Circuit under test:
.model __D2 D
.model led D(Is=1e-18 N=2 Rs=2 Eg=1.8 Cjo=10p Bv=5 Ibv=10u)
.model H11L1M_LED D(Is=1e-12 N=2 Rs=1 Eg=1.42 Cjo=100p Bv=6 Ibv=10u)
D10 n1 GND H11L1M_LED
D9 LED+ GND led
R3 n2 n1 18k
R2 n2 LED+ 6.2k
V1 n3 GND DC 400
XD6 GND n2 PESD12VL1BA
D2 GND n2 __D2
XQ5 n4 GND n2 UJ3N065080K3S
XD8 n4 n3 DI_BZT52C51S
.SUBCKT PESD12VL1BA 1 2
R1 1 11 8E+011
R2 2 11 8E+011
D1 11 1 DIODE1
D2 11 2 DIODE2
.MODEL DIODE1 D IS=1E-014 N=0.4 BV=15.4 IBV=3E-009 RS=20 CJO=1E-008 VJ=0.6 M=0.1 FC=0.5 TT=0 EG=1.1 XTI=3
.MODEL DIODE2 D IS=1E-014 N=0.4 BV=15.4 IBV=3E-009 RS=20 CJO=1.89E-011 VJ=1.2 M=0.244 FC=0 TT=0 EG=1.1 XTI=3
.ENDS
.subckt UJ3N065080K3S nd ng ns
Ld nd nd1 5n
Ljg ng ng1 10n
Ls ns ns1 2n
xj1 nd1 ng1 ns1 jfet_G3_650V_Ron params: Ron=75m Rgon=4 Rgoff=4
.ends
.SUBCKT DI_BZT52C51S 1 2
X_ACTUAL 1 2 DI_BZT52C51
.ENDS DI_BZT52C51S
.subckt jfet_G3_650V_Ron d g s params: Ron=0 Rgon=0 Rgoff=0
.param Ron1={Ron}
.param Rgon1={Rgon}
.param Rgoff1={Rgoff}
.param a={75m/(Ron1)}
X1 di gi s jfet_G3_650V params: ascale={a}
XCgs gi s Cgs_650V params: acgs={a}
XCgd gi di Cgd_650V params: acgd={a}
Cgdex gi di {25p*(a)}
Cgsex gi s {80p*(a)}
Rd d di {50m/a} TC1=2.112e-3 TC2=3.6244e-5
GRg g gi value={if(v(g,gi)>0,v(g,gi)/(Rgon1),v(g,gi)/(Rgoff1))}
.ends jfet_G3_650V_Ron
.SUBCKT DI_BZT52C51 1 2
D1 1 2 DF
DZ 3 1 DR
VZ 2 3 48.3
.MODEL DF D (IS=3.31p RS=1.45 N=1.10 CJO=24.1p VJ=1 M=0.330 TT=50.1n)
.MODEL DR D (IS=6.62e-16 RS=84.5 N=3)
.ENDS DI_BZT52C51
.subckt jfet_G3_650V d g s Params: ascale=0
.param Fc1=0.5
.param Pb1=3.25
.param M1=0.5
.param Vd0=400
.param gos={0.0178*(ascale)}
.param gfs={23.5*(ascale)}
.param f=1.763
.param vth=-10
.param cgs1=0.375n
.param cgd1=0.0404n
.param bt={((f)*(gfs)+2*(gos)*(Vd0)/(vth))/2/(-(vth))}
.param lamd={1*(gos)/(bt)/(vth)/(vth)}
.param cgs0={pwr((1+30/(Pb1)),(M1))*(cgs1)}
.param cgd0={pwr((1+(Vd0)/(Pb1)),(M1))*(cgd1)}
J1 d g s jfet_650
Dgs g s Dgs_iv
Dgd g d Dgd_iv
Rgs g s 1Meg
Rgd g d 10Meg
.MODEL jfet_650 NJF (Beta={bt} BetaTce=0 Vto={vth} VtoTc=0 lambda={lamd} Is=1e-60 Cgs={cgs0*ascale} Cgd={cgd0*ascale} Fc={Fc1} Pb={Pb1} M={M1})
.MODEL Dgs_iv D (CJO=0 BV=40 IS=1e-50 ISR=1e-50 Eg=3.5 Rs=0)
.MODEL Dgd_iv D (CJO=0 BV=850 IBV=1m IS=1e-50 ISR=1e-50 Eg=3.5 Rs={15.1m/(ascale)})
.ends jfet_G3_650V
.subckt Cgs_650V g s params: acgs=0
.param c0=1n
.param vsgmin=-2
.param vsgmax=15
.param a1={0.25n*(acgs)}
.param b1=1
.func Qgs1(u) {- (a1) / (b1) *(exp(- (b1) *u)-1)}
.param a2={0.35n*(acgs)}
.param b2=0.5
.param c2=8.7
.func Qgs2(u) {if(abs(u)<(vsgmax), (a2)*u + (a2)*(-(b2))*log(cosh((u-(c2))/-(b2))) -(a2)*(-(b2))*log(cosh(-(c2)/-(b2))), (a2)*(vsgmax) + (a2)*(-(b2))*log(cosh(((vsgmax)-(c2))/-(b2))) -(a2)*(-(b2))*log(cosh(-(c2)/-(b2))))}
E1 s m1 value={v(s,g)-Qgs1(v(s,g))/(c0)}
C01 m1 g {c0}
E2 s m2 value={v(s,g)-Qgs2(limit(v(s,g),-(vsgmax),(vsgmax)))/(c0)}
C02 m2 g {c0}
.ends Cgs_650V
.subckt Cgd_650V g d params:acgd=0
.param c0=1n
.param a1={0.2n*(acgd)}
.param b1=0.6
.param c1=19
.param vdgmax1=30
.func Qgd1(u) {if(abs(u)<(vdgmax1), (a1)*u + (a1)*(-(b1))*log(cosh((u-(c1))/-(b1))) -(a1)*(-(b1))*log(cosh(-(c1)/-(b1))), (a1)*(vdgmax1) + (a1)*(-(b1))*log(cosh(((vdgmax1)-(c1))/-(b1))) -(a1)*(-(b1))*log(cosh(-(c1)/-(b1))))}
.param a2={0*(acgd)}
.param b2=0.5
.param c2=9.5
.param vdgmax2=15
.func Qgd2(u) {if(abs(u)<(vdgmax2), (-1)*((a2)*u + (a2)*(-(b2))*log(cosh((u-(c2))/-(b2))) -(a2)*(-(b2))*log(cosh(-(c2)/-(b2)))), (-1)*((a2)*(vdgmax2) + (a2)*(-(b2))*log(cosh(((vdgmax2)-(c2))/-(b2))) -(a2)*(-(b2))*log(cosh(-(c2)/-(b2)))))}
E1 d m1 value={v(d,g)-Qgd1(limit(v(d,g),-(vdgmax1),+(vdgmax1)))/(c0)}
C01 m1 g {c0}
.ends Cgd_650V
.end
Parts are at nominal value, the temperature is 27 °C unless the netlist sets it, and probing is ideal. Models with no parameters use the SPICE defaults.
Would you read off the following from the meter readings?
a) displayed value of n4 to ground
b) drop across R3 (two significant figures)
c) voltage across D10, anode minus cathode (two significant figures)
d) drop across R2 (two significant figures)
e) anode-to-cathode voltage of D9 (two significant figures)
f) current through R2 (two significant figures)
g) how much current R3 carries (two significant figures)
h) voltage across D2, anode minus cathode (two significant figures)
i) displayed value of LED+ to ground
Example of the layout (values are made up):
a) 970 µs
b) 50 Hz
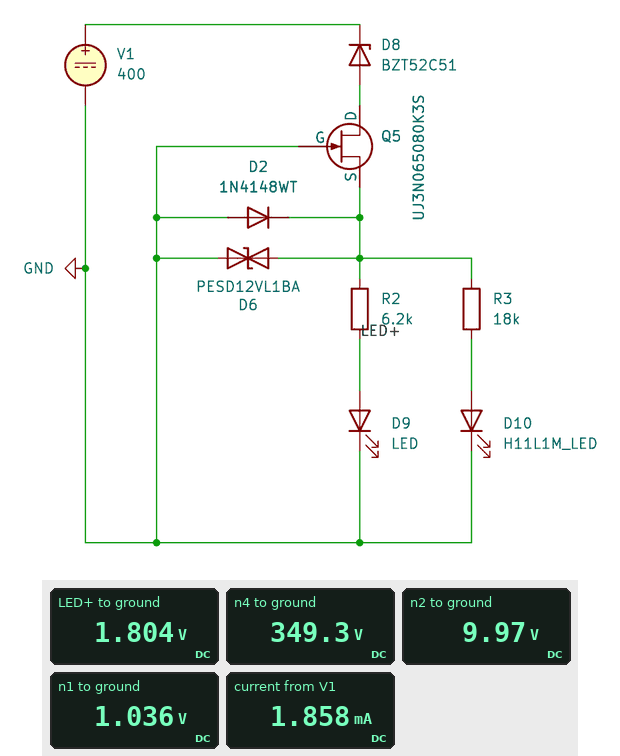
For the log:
a) 349.3 V
b) 8.9 V
c) 1.0 V
d) 8.2 V
e) 1.8 V
f) 1.3 mA
g) 500 µA
h) -10 V
i) 1.804 V
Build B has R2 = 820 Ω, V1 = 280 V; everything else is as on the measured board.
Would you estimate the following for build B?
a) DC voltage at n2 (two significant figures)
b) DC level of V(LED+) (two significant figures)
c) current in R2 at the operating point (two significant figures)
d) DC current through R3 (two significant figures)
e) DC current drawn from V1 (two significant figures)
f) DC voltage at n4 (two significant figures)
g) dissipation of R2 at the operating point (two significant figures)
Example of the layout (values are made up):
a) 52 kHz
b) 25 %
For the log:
a) 9.9 V
b) 1.9 V
c) 9.8 mA
d) 490 µA
e) 10 mA
f) 230 V
g) 78 mW
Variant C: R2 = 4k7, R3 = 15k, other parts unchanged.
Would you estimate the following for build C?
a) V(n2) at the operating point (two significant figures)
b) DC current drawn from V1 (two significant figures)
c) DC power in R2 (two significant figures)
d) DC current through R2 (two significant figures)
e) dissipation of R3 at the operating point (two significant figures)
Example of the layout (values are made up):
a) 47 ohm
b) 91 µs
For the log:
a) 10 V
b) 2.4 mA
c) 14 mW
d) 1.7 mA
e) 5.3 mW
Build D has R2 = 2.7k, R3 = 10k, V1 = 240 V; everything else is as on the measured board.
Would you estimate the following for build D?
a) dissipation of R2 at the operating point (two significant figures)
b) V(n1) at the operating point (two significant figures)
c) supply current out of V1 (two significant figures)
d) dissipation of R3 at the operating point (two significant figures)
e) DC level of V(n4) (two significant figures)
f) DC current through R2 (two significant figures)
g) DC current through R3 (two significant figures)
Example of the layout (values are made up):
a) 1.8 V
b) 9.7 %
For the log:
a) 24 mW
b) 1.1 V
c) 3.9 mA
d) 7.9 mW
e) 190 V
f) 3.0 mA
g) 890 µA
